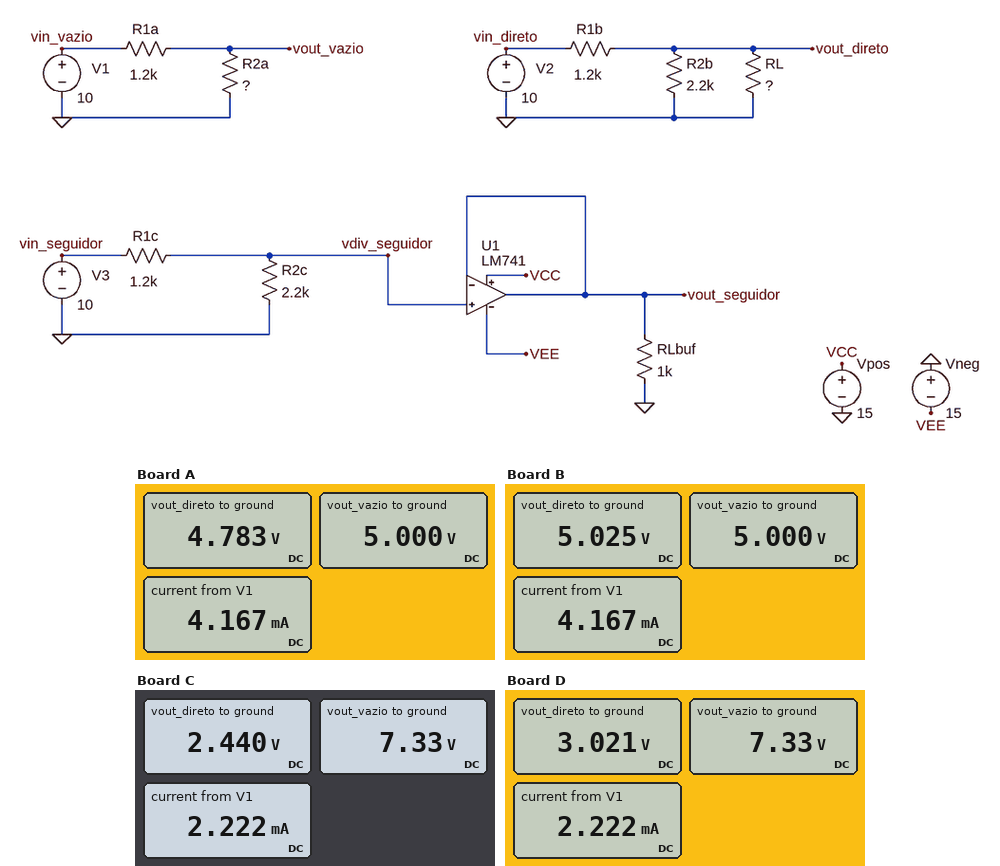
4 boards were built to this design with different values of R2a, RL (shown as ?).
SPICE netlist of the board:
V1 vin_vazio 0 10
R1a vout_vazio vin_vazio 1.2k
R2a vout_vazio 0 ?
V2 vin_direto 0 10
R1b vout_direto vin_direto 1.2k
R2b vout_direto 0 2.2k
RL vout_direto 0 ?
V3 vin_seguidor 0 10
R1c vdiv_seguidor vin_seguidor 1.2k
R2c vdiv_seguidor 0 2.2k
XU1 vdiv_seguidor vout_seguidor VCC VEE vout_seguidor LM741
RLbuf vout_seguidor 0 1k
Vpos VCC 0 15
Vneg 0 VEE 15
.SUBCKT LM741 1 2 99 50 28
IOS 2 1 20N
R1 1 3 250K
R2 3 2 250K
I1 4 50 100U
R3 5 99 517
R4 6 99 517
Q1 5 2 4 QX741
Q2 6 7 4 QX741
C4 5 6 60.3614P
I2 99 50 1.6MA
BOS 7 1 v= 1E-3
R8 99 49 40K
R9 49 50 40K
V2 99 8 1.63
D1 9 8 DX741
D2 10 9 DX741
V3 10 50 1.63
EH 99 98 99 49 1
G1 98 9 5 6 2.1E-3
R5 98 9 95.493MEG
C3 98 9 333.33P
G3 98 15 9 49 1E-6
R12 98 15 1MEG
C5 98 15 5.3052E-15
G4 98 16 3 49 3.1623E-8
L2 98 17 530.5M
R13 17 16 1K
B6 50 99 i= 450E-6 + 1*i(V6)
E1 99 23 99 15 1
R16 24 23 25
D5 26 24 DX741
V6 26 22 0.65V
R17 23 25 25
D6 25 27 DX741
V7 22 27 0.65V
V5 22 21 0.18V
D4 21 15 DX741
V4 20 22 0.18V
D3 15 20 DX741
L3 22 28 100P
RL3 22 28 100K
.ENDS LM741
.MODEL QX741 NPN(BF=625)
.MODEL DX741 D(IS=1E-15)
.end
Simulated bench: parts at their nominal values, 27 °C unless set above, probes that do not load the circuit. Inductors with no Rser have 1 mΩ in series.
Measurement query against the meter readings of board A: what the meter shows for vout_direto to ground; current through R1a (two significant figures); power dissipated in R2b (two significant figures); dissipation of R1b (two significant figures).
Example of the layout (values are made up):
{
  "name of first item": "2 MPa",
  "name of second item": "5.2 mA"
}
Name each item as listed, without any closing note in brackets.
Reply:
{
  "what the meter shows for vout_direto to ground": "4.783 V",
  "current through R1a": "4.2 mA",
  "power dissipated in R2b": "10 mW",
  "dissipation of R1b": "23 mW"
}
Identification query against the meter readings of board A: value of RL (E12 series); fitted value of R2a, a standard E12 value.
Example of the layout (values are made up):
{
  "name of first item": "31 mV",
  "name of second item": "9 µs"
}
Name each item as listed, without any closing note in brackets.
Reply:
{
  "value of RL": "2.2 kΩ",
  "fitted value of R2a, a standard E12 value": "1.2 kΩ"
}
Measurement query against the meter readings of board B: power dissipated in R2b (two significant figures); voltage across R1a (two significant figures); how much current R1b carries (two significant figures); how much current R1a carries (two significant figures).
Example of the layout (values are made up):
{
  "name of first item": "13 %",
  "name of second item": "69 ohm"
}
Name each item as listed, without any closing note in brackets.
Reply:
{
  "power dissipated in R2b": "11 mW",
  "voltage across R1a": "5.0 V",
  "how much current R1b carries": "4.1 mA",
  "how much current R1a carries": "4.2 mA"
}
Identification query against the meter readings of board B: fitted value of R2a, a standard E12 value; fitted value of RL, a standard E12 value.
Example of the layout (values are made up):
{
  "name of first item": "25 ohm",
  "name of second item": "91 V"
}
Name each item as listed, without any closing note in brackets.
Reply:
{
  "fitted value of R2a, a standard E12 value": "1.2 kΩ",
  "fitted value of RL, a standard E12 value": "2.7 kΩ"
}
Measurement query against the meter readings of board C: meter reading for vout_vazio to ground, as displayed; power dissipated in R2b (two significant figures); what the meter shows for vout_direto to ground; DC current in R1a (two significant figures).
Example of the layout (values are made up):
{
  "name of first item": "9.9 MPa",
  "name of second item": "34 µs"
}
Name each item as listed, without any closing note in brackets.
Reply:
{
  "meter reading for vout_vazio to ground, as displayed": "7.33 V",
  "power dissipated in R2b": "2.7 mW",
  "what the meter shows for vout_direto to ground": "2.440 V",
  "DC current in R1a": "2.2 mA"
}
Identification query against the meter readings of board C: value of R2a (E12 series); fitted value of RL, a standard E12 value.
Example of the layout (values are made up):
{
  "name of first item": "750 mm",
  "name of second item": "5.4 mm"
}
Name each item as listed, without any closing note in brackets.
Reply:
{
  "value of R2a": "3.3 kΩ",
  "fitted value of RL, a standard E12 value": "470 Ω"
}
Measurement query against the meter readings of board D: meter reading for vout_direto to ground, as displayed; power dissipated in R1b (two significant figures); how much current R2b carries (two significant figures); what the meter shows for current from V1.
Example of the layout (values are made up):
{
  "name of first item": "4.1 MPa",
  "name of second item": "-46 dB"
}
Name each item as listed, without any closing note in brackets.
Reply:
{
  "meter reading for vout_direto to ground, as displayed": "3.021 V",
  "power dissipated in R1b": "41 mW",
  "how much current R2b carries": "1.4 mA",
  "what the meter shows for current from V1": "2.222 mA"
}
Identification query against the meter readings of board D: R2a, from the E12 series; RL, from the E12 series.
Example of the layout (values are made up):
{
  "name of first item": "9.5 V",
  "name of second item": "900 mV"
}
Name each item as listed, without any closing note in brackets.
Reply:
{
  "R2a, from the E12 series": "3.3 kΩ",
  "RL, from the E12 series": "680 Ω"
}
